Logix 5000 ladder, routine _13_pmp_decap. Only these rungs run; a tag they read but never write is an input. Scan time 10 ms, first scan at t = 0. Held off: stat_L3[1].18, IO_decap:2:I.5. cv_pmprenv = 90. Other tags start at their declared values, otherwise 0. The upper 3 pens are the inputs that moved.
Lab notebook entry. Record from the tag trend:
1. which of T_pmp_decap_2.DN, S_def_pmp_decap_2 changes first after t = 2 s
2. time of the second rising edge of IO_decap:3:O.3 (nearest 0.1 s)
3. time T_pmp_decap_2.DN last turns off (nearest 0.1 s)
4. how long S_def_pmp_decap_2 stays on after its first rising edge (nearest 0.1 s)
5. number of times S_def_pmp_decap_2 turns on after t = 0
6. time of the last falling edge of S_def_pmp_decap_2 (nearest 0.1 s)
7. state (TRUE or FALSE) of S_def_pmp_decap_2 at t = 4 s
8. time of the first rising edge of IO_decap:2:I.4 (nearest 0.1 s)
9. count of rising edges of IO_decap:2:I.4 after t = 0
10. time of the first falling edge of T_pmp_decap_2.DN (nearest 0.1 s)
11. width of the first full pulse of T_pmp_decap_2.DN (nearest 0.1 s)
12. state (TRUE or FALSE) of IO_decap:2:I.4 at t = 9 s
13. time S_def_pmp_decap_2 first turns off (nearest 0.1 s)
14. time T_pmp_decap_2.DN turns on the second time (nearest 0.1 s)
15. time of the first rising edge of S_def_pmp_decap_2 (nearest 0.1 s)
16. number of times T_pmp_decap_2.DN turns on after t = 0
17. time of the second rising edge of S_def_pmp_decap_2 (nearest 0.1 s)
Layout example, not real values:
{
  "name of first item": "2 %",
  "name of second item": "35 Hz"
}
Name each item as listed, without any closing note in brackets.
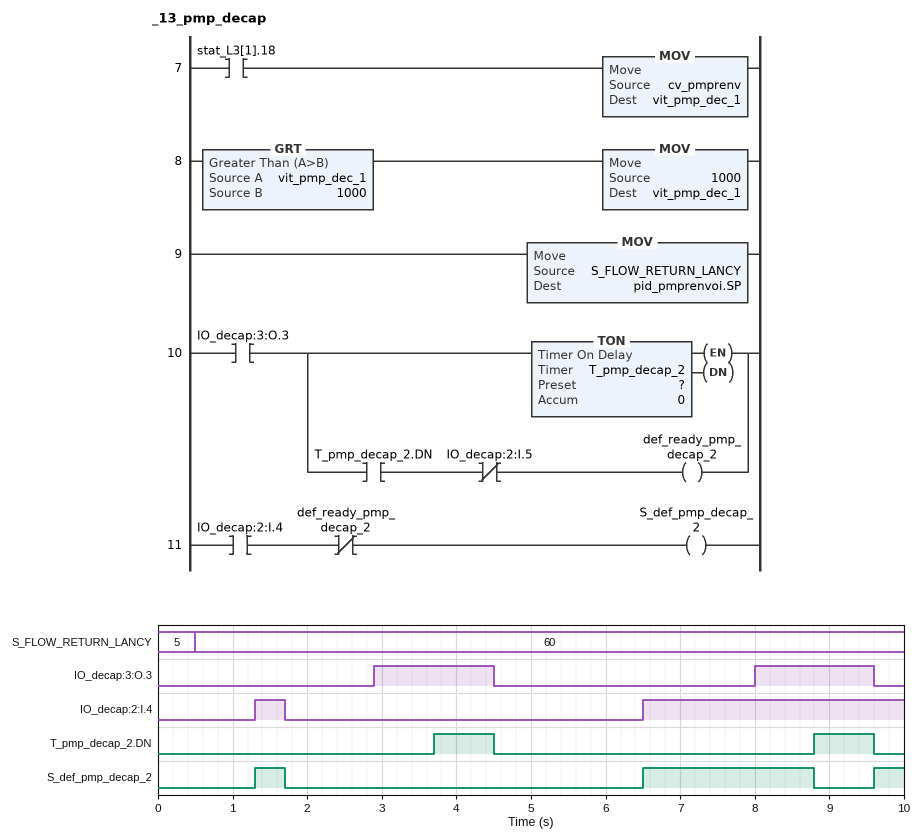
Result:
{
  "which of T_pmp_decap_2.DN, S_def_pmp_decap_2 changes first after t = 2 s": "T_pmp_decap_2.DN",
  "time of the second rising edge of IO_decap:3:O.3": "8.0 s",
  "time T_pmp_decap_2.DN last turns off": "9.6 s",
  "how long S_def_pmp_decap_2 stays on after its first rising edge": "0.4 s",
  "number of times S_def_pmp_decap_2 turns on after t = 0": "3",
  "time of the last falling edge of S_def_pmp_decap_2": "8.8 s",
  "state (TRUE or FALSE) of S_def_pmp_decap_2 at t = 4 s": "FALSE",
  "time of the first rising edge of IO_decap:2:I.4": "1.3 s",
  "count of rising edges of IO_decap:2:I.4 after t = 0": "2",
  "time of the first falling edge of T_pmp_decap_2.DN": "4.5 s",
  "width of the first full pulse of T_pmp_decap_2.DN": "0.8 s",
  "state (TRUE or FALSE) of IO_decap:2:I.4 at t = 9 s": "TRUE",
  "time S_def_pmp_decap_2 first turns off": "1.7 s",
  "time T_pmp_decap_2.DN turns on the second time": "8.8 s",
  "time of the first rising edge of S_def_pmp_decap_2": "1.3 s",
  "number of times T_pmp_decap_2.DN turns on after t = 0": "2",
  "time of the second rising edge of S_def_pmp_decap_2": "6.5 s"
}
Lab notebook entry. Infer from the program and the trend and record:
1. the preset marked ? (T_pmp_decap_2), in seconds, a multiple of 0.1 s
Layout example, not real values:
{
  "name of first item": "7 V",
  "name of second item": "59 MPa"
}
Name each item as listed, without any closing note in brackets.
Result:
{
  "the preset marked ? (T_pmp_decap_2), in seconds, a multiple of 0.1 s": "0.8 s"
}
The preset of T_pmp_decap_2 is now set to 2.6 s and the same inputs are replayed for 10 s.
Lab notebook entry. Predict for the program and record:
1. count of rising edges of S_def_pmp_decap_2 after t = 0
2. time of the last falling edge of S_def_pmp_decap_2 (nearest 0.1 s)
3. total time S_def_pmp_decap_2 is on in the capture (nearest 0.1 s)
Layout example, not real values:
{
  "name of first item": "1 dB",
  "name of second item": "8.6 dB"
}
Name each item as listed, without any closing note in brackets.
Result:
{
  "count of rising edges of S_def_pmp_decap_2 after t = 0": "2",
  "time of the last falling edge of S_def_pmp_decap_2": "1.7 s",
  "total time S_def_pmp_decap_2 is on in the capture": "3.9 s"
}
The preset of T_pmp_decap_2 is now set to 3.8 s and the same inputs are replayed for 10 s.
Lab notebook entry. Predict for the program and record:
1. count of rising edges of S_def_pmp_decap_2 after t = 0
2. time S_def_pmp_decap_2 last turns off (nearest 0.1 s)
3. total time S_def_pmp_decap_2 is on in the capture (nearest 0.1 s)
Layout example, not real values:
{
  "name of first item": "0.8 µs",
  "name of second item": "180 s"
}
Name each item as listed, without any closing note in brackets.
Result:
{
  "count of rising edges of S_def_pmp_decap_2 after t = 0": "2",
  "time S_def_pmp_decap_2 last turns off": "1.7 s",
  "total time S_def_pmp_decap_2 is on in the capture": "3.9 s"
}
